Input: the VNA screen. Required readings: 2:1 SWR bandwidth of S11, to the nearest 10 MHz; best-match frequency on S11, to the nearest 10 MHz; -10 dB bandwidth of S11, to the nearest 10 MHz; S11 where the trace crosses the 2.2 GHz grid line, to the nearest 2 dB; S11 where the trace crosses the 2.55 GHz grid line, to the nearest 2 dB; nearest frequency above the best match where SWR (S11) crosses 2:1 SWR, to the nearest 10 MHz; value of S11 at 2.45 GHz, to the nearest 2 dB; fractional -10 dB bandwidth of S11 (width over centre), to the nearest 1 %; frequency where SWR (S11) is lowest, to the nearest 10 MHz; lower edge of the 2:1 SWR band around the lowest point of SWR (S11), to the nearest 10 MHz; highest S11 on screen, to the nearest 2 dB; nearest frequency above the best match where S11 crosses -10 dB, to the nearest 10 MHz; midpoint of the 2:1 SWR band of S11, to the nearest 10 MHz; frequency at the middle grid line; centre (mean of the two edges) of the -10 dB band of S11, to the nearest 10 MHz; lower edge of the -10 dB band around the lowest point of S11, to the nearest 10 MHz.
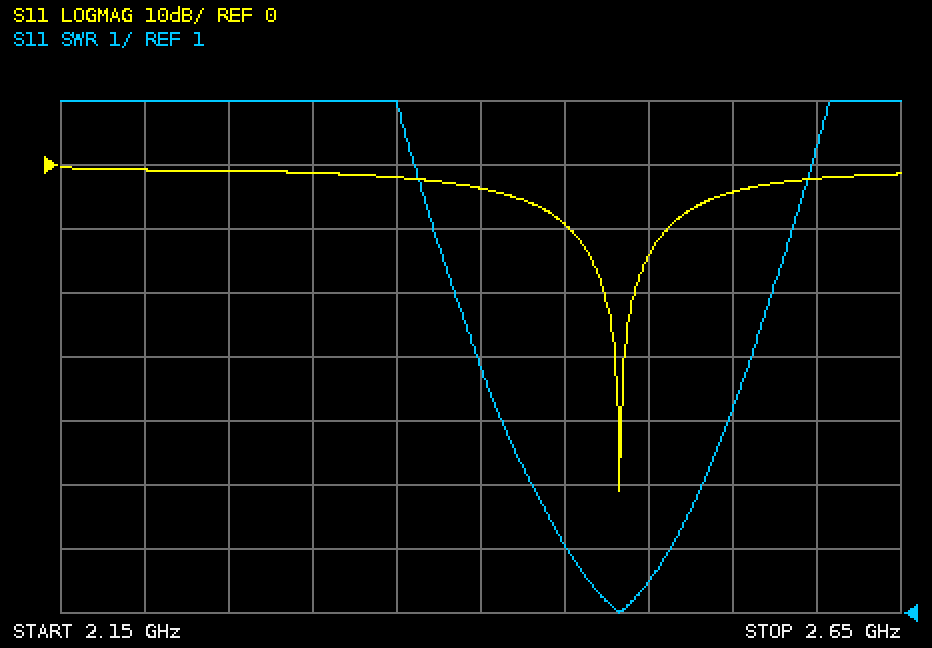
60 MHz
2.48 GHz
60 MHz
0 dB
-4 dB
2.51 GHz
-10 dB
2 %
2.48 GHz
2.45 GHz
0 dB
2.51 GHz
2.48 GHz
2.4 GHz
2.48 GHz
2.45 GHz
